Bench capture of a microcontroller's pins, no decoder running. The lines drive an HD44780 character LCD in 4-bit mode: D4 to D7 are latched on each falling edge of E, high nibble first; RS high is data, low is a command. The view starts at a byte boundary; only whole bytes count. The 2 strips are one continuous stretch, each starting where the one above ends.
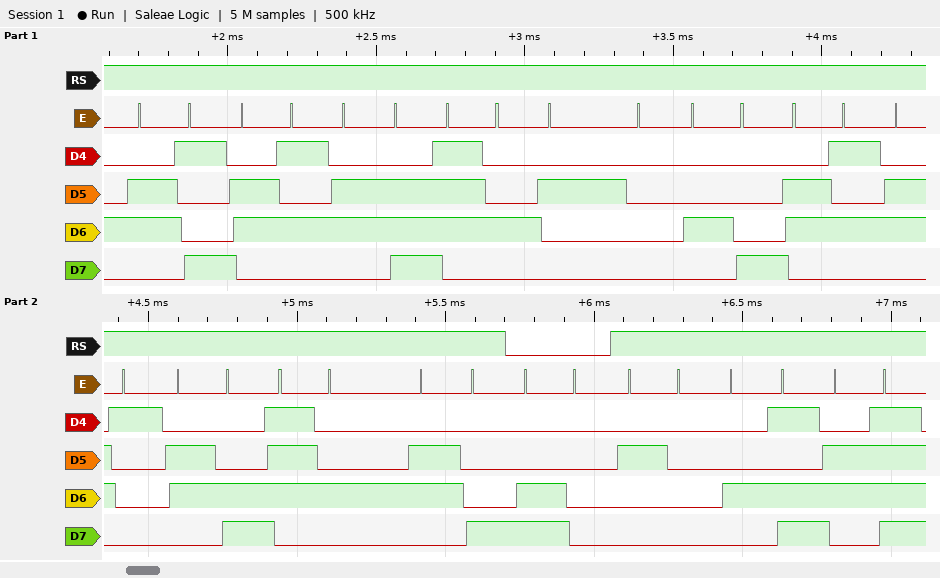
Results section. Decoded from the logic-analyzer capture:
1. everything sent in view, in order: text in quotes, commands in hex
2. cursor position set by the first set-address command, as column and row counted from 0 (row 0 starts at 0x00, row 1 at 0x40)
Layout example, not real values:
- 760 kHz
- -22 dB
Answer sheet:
- "ient Health" 0xC0 " Mo"
- column 0, row 1
